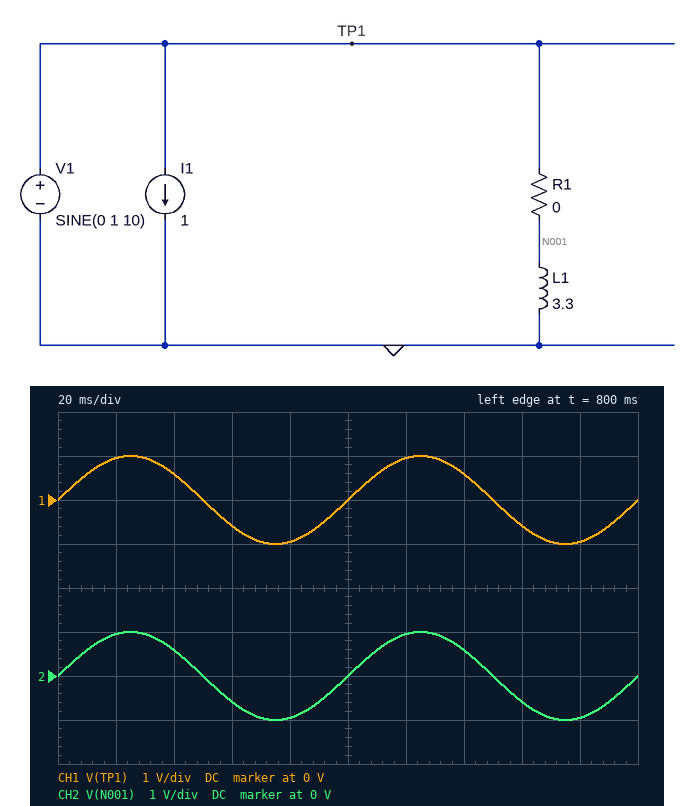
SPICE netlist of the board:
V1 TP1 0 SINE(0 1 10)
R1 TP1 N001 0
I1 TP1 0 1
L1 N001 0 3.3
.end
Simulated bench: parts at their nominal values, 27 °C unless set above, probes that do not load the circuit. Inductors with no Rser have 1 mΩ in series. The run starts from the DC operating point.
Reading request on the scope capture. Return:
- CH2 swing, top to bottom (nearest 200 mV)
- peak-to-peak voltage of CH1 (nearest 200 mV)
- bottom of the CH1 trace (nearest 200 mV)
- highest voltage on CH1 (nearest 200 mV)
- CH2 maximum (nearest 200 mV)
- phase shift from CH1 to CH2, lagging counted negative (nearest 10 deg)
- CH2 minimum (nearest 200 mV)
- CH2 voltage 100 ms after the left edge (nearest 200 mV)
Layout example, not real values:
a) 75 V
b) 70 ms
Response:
a) 2.0 V
b) 2.0 V
c) -1.0 V
d) 1.0 V
e) 1.0 V
f) 0 deg
g) -1.0 V
h) 0 V
